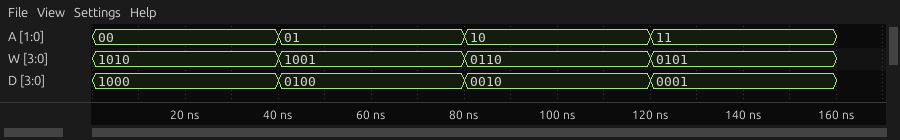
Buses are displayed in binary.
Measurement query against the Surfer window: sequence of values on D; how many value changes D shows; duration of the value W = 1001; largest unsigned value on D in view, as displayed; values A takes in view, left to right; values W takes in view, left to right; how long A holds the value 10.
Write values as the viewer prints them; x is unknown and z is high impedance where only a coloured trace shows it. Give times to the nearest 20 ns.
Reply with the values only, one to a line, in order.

1000, 0100, 0010, 0001
3
40 ns
1000
00, 01, 10, 11
1010, 1001, 0110, 0101
40 ns
